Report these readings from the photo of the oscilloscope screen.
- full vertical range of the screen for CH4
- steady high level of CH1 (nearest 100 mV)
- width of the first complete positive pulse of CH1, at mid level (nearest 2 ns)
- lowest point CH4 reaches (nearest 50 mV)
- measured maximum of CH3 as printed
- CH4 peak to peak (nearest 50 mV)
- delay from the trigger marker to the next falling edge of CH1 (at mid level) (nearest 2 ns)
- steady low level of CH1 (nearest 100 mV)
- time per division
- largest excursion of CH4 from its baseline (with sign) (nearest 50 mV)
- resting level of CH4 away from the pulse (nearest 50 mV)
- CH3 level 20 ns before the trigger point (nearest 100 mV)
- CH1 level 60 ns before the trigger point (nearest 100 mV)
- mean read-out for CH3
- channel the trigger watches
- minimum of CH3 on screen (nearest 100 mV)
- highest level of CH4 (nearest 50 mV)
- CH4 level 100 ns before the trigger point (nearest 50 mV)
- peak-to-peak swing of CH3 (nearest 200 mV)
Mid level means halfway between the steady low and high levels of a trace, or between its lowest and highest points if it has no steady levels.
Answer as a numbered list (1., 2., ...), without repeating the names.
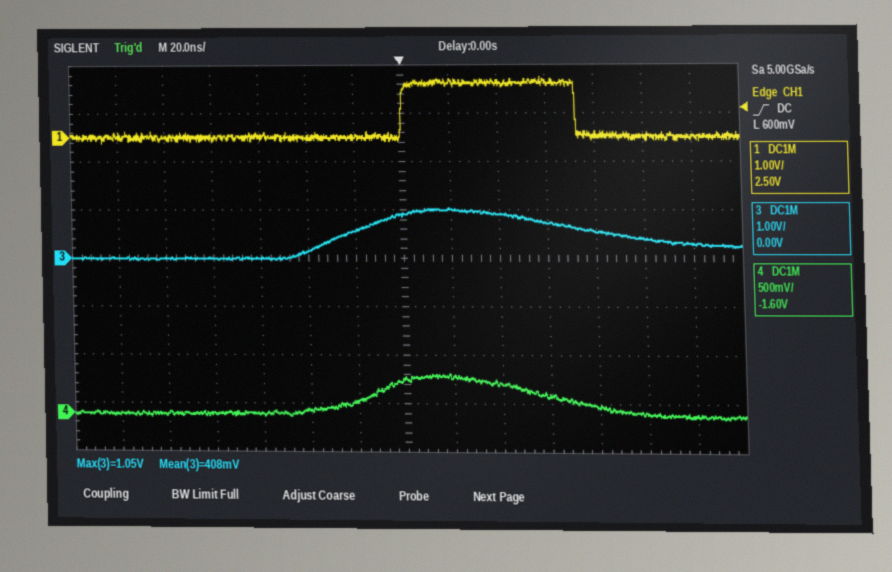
1. 4 V
2. 1.1 V
3. 72 ns
4. -50 mV
5. 1.05 V
6. 450 mV
7. 72 ns
8. 0.0 V
9. 20 ns
10. +400 mV
11. 0 mV
12. 600 mV
13. 0.0 V
14. 408 mV
15. CH1
16. 0.0 V
17. 400 mV
18. 0 mV
19. 1.0 V
